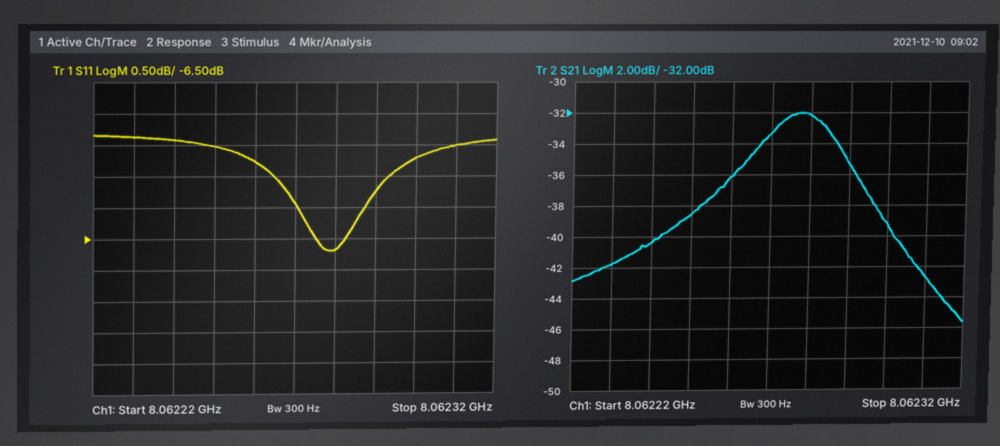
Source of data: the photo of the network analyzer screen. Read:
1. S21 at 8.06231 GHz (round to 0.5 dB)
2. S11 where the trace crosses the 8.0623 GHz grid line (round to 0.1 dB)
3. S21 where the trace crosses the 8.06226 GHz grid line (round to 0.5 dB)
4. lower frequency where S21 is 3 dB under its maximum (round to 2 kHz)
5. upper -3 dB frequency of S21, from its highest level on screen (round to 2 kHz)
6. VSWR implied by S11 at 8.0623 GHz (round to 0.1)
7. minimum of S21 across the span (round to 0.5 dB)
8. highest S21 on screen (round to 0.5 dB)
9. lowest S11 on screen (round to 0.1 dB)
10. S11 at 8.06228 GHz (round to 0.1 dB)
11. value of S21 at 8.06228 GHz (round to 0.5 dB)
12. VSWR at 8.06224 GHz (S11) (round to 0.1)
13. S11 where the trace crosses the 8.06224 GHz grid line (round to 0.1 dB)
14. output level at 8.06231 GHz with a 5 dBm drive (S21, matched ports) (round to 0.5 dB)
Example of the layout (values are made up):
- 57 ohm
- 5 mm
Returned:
- -42.5 dB
- -5.2 dB
- -36.0 dB
- 8.062264 GHz
- 8.062290 GHz
- 3.4
- -45.5 dB
- -32.0 dB
- -6.7 dB
- -6.7 dB
- -32.0 dB
- 3.6
- -4.9 dB
- -37.5 dBm
